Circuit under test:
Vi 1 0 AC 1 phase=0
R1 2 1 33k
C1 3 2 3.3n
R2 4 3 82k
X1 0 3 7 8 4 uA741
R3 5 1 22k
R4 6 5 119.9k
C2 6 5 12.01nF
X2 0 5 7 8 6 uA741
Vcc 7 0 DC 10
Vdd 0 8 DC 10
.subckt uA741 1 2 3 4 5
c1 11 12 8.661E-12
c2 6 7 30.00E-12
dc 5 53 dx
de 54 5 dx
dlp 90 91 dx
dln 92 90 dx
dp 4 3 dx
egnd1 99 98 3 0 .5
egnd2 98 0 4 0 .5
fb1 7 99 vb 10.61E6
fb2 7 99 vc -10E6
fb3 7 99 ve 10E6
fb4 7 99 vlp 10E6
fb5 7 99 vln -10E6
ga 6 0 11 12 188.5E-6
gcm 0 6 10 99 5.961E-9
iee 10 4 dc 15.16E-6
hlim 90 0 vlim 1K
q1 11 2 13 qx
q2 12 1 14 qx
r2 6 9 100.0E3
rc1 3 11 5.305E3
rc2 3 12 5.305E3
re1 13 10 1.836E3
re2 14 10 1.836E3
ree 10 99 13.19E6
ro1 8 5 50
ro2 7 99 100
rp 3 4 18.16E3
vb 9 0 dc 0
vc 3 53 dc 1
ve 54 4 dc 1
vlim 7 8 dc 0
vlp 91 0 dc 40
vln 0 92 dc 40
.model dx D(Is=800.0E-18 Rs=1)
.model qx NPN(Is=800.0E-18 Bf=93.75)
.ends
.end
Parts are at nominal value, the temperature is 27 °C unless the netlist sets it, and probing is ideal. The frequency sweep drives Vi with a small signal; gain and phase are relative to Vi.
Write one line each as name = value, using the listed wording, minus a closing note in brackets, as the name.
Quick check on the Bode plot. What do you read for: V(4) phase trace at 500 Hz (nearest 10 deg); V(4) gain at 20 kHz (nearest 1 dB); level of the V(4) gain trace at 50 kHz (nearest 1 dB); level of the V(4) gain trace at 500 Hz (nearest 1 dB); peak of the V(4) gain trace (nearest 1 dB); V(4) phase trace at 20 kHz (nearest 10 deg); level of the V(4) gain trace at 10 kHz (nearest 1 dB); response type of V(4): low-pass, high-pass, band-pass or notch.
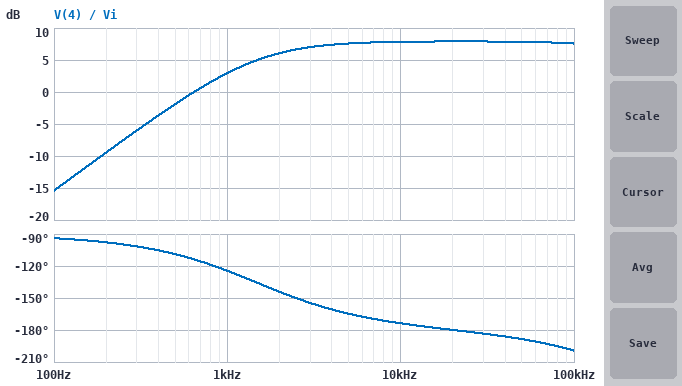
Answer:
V(4) phase trace at 500 Hz = -110 deg
V(4) gain at 20 kHz = 8 dB
level of the V(4) gain trace at 50 kHz = 8 dB
level of the V(4) gain trace at 500 Hz = -2 dB
peak of the V(4) gain trace = 8 dB
V(4) phase trace at 20 kHz = -180 deg
level of the V(4) gain trace at 10 kHz = 8 dB
response type of V(4): low-pass, high-pass, band-pass or notch = high-pass
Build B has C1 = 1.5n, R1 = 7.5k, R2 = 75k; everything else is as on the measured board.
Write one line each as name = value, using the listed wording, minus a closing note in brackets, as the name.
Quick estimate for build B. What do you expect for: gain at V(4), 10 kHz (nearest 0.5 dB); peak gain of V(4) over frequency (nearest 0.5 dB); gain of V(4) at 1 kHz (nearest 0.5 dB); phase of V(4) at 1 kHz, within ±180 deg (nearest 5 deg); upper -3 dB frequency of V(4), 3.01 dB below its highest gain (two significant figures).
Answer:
gain at V(4), 10 kHz = 15.5 dB
peak gain of V(4) over frequency = 20.0 dB
gain of V(4) at 1 kHz = -3.0 dB
phase of V(4) at 1 kHz, within ±180 deg = -95 deg
upper -3 dB frequency of V(4), 3.01 dB below its highest gain = 110 kHz
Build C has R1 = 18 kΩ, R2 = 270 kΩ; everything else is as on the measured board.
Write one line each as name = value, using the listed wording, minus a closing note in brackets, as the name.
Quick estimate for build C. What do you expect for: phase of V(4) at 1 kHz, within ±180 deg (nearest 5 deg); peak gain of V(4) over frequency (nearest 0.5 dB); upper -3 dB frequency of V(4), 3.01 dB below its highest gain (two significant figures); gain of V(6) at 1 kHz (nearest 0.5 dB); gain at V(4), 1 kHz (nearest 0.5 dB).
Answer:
phase of V(4) at 1 kHz, within ±180 deg = -110 deg
peak gain of V(4) over frequency = 23.5 dB
upper -3 dB frequency of V(4), 3.01 dB below its highest gain = 66 kHz
gain of V(6) at 1 kHz = -4.5 dB
gain at V(4), 1 kHz = 14.5 dB
